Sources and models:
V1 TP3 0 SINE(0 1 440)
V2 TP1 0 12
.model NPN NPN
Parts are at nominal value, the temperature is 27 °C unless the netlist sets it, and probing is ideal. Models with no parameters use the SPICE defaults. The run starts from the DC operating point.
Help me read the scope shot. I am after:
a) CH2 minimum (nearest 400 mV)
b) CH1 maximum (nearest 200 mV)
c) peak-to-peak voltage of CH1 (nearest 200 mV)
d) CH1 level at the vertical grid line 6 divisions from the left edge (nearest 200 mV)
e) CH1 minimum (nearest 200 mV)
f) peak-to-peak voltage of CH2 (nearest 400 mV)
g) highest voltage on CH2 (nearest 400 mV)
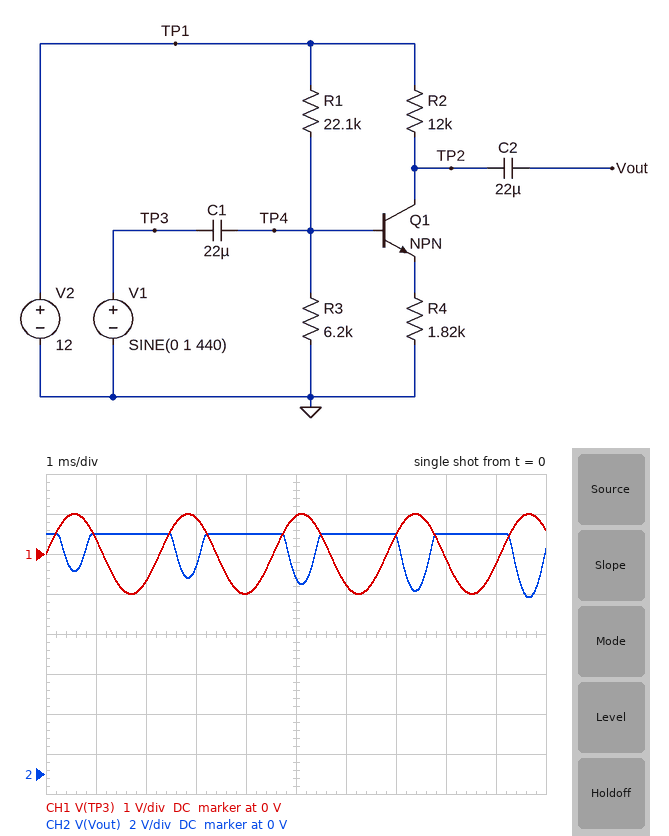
8.8 V
1.0 V
2.0 V
-800 mV
-1.0 V
3.2 V
12.0 V
